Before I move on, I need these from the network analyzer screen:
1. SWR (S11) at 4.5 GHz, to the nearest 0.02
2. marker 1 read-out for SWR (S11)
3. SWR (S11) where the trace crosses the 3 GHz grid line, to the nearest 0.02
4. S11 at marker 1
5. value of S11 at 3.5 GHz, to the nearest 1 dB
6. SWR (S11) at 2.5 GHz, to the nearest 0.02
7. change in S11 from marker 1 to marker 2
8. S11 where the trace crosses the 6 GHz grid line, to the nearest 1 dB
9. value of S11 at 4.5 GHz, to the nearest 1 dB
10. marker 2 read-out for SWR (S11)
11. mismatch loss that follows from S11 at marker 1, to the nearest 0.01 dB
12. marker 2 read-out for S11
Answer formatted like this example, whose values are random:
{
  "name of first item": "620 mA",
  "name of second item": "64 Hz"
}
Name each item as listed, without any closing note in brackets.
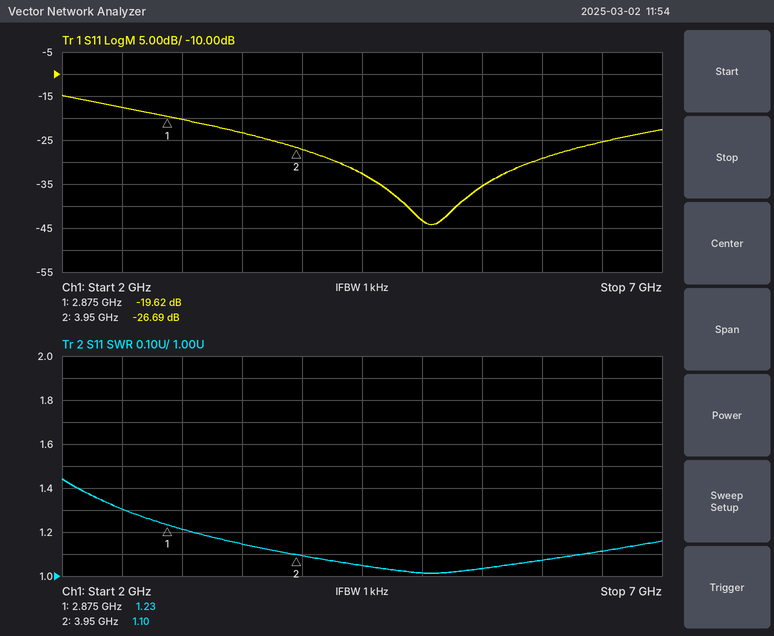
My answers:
{
  "SWR (S11) at 4.5 GHz, to the nearest 0.02": "1.04",
  "marker 1 read-out for SWR": "1.23",
  "SWR (S11) where the trace crosses the 3 GHz grid line, to the nearest 0.02": "1.22",
  "S11 at marker 1": "-19.62 dB",
  "value of S11 at 3.5 GHz, to the nearest 1 dB": "-23 dB",
  "SWR (S11) at 2.5 GHz, to the nearest 0.02": "1.30",
  "change in S11 from marker 1 to marker 2": "-7.07 dB",
  "S11 where the trace crosses the 6 GHz grid line, to the nearest 1 dB": "-29 dB",
  "value of S11 at 4.5 GHz, to the nearest 1 dB": "-33 dB",
  "marker 2 read-out for SWR": "1.10",
  "mismatch loss that follows from S11 at marker 1, to the nearest 0.01 dB": "0.05 dB",
  "marker 2 read-out for S11": "-26.69 dB"
}
